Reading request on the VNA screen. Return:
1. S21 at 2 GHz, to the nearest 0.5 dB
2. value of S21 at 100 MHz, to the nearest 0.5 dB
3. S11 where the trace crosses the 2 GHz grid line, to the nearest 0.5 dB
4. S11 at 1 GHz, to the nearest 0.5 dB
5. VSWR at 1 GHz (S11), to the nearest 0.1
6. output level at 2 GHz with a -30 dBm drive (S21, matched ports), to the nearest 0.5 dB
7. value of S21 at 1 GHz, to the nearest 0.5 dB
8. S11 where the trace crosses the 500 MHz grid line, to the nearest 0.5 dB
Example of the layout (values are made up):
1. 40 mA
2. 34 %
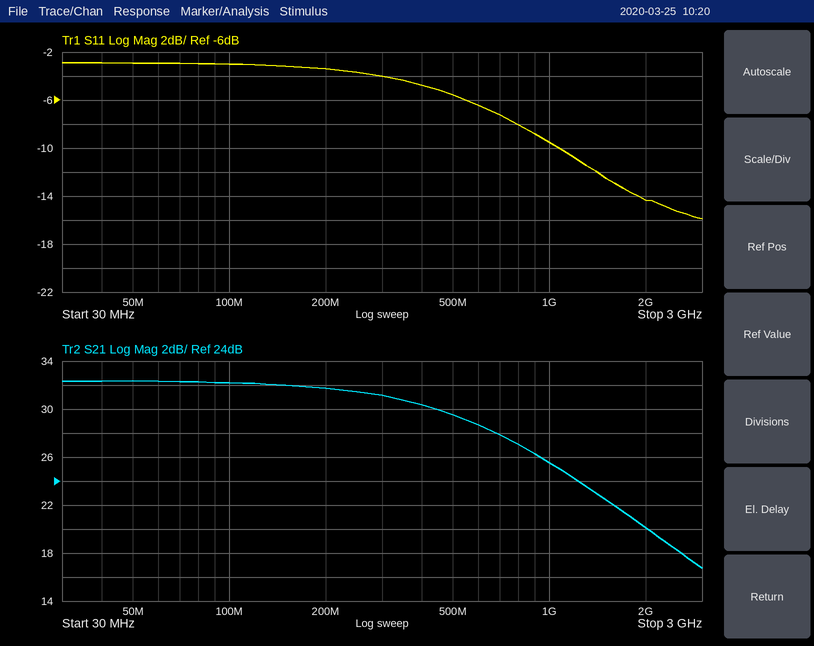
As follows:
1. 20.0 dB
2. 32.0 dB
3. -14.5 dB
4. -9.5 dB
5. 2.0
6. -10.0 dBm
7. 25.5 dB
8. -5.5 dB
